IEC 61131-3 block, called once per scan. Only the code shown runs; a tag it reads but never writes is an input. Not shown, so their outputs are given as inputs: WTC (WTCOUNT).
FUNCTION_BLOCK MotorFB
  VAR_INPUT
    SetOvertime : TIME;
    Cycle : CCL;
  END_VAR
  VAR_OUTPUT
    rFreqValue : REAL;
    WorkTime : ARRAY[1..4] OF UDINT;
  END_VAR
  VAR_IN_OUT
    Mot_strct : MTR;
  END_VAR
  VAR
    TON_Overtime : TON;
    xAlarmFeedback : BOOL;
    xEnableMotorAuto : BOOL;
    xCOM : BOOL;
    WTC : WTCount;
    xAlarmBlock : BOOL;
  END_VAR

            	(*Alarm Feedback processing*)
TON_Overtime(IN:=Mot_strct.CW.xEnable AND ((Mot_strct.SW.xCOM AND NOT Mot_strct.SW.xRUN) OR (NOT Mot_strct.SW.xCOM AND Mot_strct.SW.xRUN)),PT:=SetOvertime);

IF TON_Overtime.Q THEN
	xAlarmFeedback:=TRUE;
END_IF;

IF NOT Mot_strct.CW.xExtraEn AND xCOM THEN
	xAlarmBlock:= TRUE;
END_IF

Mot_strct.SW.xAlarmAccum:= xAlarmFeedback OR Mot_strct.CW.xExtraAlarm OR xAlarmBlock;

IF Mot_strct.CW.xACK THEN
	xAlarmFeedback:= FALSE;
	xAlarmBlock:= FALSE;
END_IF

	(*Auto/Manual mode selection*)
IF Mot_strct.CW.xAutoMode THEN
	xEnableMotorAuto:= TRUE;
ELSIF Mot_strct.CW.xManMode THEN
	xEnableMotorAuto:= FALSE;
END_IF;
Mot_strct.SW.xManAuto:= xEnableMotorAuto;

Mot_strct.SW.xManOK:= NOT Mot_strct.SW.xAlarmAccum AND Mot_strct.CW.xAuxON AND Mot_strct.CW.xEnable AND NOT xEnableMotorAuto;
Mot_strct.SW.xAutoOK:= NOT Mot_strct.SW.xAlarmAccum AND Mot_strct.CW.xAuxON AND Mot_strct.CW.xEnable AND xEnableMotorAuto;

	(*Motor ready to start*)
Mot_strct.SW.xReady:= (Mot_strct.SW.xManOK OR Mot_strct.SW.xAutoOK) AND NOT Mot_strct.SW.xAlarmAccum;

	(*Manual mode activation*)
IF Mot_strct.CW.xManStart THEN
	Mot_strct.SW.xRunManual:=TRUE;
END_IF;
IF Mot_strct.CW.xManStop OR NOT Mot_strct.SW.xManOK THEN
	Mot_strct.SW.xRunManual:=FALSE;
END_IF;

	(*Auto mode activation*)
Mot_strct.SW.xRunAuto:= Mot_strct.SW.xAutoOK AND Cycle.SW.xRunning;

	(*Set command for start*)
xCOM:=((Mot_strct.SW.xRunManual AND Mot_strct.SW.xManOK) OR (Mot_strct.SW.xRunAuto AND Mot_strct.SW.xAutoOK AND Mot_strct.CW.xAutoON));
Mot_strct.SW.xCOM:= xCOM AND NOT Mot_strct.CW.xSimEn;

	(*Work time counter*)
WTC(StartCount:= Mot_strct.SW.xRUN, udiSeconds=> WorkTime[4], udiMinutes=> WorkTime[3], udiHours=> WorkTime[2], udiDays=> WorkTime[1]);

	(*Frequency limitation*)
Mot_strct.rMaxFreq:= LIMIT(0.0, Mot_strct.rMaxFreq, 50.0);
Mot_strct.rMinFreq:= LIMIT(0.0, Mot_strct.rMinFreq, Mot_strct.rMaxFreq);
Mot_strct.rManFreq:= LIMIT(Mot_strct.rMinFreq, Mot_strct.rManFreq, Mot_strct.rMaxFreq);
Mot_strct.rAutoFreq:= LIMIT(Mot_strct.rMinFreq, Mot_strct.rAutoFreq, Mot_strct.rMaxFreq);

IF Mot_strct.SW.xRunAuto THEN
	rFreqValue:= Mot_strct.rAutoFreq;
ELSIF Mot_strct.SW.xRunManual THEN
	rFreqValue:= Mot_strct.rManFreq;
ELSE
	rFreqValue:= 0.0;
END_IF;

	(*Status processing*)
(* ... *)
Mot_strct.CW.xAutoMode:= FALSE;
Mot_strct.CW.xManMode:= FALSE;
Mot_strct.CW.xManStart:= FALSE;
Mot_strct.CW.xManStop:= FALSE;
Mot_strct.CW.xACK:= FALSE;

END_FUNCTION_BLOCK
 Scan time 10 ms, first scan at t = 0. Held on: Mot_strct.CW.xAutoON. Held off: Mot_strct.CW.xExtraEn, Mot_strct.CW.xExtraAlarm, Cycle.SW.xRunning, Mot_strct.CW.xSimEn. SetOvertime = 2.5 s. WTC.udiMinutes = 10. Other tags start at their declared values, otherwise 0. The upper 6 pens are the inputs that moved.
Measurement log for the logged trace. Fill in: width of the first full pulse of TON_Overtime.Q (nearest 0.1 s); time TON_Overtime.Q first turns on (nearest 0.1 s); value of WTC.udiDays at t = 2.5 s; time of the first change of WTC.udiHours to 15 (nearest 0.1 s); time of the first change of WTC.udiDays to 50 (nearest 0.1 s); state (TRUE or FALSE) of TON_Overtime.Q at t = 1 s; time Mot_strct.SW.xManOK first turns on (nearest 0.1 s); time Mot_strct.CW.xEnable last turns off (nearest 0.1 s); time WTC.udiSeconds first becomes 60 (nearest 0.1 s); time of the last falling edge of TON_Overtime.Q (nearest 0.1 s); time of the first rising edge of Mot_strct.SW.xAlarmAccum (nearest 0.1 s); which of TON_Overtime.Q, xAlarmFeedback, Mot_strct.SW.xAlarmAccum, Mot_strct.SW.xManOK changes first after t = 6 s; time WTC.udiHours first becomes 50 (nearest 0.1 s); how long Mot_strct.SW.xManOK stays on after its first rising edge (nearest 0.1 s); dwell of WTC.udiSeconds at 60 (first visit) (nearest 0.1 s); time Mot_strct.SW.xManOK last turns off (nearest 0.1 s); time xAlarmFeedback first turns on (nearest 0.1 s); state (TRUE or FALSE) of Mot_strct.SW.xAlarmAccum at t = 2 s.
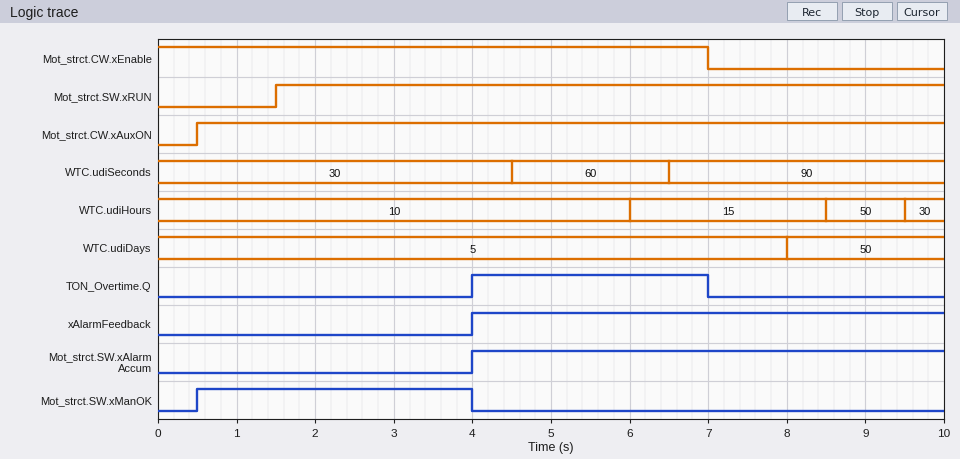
3.0 s
4.0 s
5
6.0 s
8.0 s
FALSE
0.5 s
7.0 s
4.5 s
7.0 s
4.0 s
TON_Overtime.Q
8.5 s
3.5 s
2.0 s
4.0 s
4.0 s
FALSE
